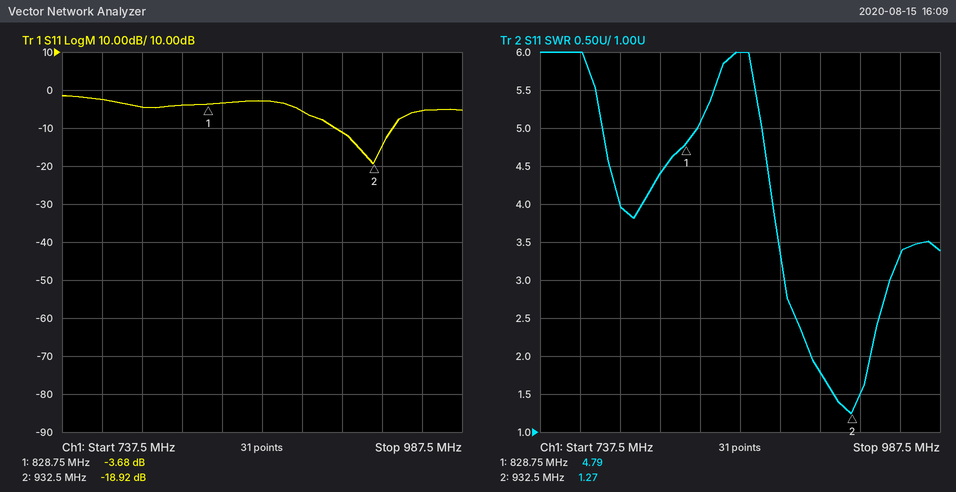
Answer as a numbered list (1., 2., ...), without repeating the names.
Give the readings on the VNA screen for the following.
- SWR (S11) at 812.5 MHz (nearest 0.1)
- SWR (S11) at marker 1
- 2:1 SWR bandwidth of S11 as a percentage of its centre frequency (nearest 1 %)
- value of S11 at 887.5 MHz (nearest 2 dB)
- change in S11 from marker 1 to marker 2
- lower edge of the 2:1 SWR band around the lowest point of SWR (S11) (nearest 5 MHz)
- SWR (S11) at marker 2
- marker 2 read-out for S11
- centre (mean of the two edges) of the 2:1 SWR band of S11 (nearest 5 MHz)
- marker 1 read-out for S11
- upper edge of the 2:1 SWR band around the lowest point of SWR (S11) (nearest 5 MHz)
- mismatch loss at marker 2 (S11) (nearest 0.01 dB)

1. 4.4
2. 4.79
3. 4 %
4. -6 dB
5. -15.24 dB
6. 905 MHz
7. 1.27
8. -18.92 dB
9. 925 MHz
10. -3.68 dB
11. 945 MHz
12. 0.06 dB
